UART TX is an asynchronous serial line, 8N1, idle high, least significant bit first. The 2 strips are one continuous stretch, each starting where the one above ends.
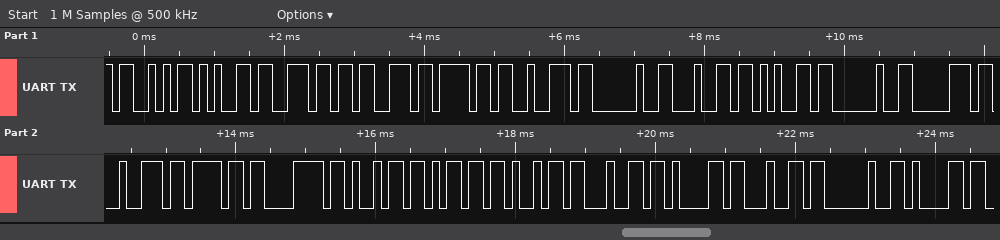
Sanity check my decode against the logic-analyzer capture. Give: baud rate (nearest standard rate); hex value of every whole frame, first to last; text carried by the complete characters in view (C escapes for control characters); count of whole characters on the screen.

9600 baud
53 65 6E 73 6F 72 20 64 65 20 70 72 6F 78 69 6D 69 64 61 64 20 61
"Sensor de proximidad a"
22
